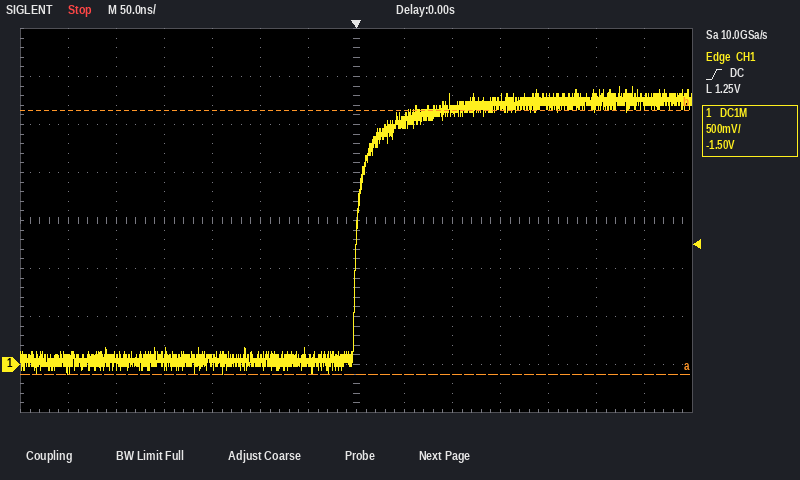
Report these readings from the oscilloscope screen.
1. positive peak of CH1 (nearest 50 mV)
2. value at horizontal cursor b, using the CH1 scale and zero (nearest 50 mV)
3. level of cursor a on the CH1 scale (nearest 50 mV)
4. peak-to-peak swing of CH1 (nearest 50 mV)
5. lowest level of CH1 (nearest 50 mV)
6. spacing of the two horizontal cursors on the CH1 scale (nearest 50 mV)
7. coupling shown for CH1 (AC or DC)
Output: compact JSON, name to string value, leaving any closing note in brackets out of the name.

{"positive peak of CH1": "2.90 V", "value at horizontal cursor b, using the CH1 scale and zero": "2.65 V", "level of cursor a on the CH1 scale": "-100 mV", "peak-to-peak swing of CH1": "3.00 V", "lowest level of CH1": "-100 mV", "spacing of the two horizontal cursors on the CH1 scale": "2.75 V", "coupling shown for CH1": "DC"}
